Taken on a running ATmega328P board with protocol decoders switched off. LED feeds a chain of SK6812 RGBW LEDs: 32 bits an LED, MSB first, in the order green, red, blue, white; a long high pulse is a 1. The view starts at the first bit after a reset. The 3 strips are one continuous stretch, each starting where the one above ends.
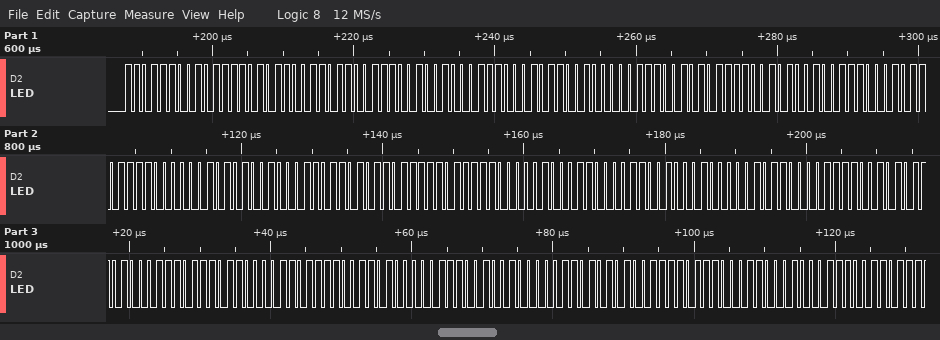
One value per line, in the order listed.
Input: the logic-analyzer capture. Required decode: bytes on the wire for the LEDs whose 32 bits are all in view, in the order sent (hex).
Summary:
DC BD 66 CE 48 E2 C8 39 5E 52 71 6F 02 A4 6D 6F BE 08 C3 22 0B 0F 2B 47 76 1B CD 07 24 1A A7 B8
